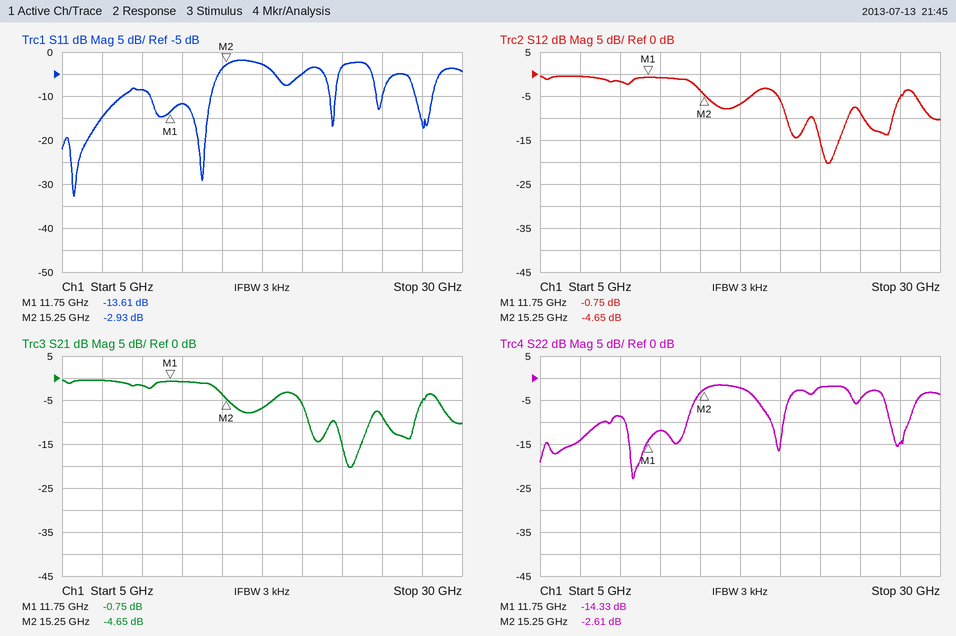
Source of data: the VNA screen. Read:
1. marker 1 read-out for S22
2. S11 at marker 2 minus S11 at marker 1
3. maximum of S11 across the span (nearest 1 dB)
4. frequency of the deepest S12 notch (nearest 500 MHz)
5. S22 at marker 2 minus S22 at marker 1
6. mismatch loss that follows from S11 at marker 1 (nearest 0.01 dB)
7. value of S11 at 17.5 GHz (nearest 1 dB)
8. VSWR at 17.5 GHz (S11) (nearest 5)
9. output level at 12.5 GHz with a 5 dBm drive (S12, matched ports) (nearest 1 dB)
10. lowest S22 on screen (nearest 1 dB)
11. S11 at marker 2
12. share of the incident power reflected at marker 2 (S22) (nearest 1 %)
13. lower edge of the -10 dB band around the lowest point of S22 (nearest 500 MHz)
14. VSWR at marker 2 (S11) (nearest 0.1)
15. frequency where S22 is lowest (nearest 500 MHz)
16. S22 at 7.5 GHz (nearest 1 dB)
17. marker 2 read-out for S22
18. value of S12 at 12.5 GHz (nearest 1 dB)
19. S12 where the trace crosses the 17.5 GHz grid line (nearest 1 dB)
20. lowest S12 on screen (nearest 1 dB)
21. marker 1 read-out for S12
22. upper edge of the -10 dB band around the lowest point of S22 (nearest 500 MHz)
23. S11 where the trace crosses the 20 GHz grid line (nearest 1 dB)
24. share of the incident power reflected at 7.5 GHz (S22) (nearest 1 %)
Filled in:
-14.33 dB
10.68 dB
-2 dB
23.0 GHz
11.72 dB
0.19 dB
-3 dB
5
4 dBm
-23 dB
-2.93 dB
55 %
10.5 GHz
6.0
11.0 GHz
-14 dB
-2.61 dB
-1 dB
-7 dB
-20 dB
-0.75 dB
14.0 GHz
-5 dB
4 %
